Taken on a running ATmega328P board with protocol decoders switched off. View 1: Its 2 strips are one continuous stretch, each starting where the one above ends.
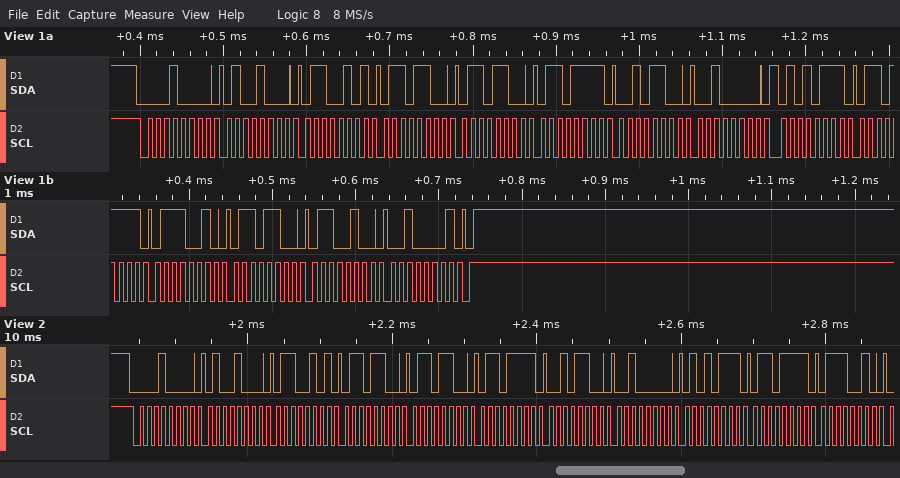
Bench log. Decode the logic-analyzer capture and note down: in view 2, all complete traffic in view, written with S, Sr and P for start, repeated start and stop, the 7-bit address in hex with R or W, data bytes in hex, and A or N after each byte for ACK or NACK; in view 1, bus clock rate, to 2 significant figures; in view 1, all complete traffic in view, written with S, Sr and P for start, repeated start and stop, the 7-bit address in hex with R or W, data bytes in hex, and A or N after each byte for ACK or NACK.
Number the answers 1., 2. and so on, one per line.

1. S 08W A 48 A 65 A 6C A 6C A 6F A 2C A 20 A 57 A 6F A 72 A
2. 100 kHz
3. S 08W A 48 A 65 A 6C A 6C A 6F A 2C A 20 A 57 A 6F A 72 A 6C A 64 A 21 A P
